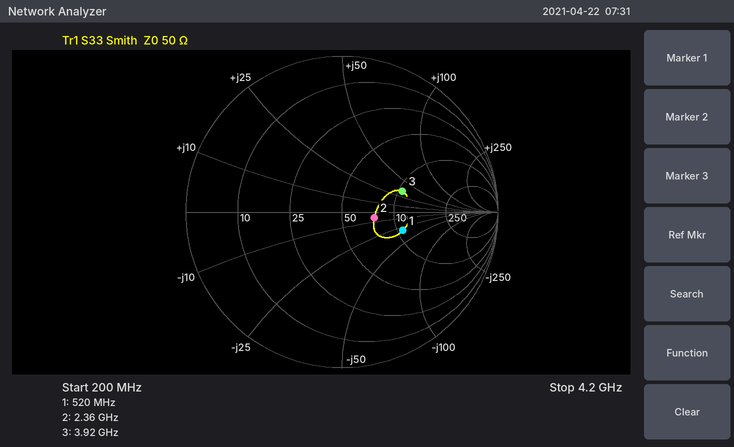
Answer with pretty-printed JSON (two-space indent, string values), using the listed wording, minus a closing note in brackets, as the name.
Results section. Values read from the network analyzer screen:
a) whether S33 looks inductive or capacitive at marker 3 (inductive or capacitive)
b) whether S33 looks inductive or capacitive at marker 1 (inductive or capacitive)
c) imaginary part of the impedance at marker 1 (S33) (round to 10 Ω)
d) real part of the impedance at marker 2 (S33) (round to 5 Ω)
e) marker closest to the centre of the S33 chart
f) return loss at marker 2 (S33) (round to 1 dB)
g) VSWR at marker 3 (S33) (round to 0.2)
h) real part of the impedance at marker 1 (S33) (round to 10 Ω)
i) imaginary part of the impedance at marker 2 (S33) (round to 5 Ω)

{
  "whether S33 looks inductive or capacitive at marker 3": "inductive",
  "whether S33 looks inductive or capacitive at marker 1": "capacitive",
  "imaginary part of the impedance at marker 1 (S33)": "-30 Ω",
  "real part of the impedance at marker 2 (S33)": "75 Ω",
  "marker closest to the centre of the S33 chart": "marker 2",
  "return loss at marker 2 (S33)": "14 dB",
  "VSWR at marker 3 (S33)": "2.4",
  "real part of the impedance at marker 1 (S33)": "110 Ω",
  "imaginary part of the impedance at marker 2 (S33)": "-5 Ω"
}
